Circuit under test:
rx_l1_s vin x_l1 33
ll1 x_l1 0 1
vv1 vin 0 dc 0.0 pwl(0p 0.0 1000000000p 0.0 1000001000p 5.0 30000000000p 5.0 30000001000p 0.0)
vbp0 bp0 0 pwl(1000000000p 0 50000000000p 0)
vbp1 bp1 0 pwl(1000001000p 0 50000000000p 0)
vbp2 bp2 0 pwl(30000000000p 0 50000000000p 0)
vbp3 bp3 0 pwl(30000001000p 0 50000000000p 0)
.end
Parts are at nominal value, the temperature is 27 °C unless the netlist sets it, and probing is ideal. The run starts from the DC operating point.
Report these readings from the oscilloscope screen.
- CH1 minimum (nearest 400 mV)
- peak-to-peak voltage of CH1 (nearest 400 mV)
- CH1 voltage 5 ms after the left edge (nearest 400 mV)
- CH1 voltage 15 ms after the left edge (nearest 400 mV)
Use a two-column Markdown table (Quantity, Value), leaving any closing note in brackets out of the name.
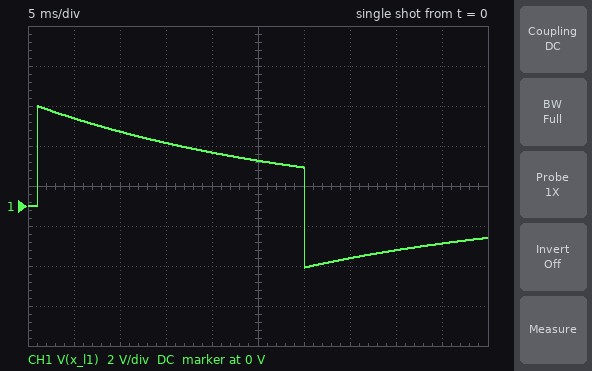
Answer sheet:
| Quantity | Value |
|---|---|
| CH1 minimum | -3.2 V |
| peak-to-peak voltage of CH1 | 8.0 V |
| CH1 voltage 5 ms after the left edge | 4.4 V |
| CH1 voltage 15 ms after the left edge | 3.2 V |
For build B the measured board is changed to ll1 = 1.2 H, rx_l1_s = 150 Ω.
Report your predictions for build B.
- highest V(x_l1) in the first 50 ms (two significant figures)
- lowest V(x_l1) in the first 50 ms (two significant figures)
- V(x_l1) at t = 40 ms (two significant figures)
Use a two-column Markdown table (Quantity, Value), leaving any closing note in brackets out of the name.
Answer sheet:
| Quantity | Value |
|---|---|
| highest V(x_l1) in the first 50 ms | 5.0 V |
| lowest V(x_l1) in the first 50 ms | -4.9 V |
| V(x_l1) at t = 40 ms | -1.4 V |
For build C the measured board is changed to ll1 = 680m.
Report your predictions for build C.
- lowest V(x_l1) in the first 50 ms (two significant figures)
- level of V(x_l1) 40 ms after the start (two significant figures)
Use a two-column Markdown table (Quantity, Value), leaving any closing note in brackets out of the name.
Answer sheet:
| Quantity | Value |
|---|---|
| lowest V(x_l1) in the first 50 ms | -3.8 V |
| level of V(x_l1) 40 ms after the start | -2.3 V |
